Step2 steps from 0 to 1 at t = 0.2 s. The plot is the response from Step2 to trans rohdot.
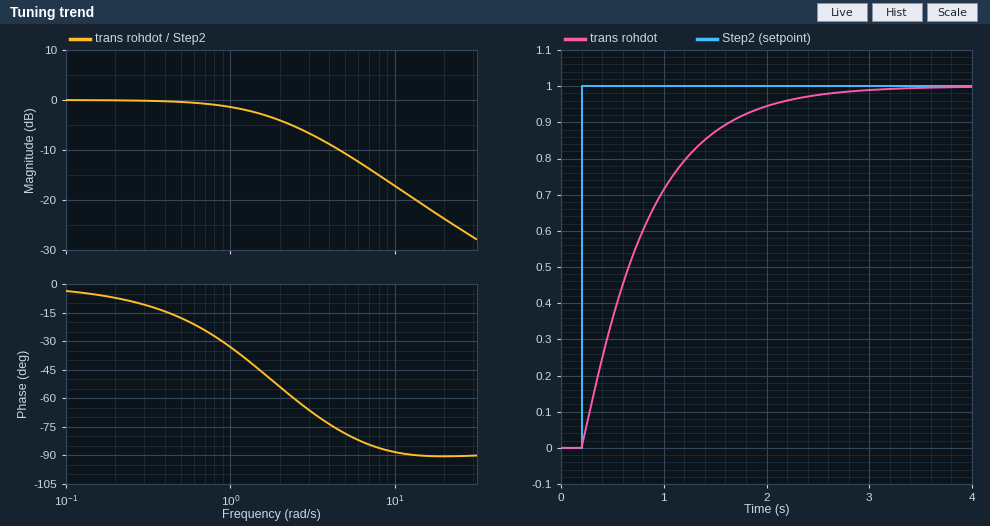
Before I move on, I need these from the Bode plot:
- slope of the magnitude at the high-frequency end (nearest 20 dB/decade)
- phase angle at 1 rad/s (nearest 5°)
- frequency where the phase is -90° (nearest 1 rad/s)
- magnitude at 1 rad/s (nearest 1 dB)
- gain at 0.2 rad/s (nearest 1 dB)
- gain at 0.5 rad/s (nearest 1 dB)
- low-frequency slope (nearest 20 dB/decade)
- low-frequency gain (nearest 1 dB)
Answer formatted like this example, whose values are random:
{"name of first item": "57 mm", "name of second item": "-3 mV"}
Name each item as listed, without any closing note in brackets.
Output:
{"slope of the magnitude at the high-frequency end": "-20 dB/decade", "phase angle at 1 rad/s": "-35°", "frequency where the phase is -90°": "14 rad/s", "magnitude at 1 rad/s": "-1 dB", "gain at 0.2 rad/s": "0 dB", "gain at 0.5 rad/s": "0 dB", "low-frequency slope": "0 dB/decade", "low-frequency gain": "0 dB"}
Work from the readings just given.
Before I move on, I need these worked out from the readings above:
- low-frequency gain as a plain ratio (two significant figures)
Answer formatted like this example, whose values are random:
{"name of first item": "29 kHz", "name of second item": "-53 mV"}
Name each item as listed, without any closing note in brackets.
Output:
{"low-frequency gain as a plain ratio": "1.0"}
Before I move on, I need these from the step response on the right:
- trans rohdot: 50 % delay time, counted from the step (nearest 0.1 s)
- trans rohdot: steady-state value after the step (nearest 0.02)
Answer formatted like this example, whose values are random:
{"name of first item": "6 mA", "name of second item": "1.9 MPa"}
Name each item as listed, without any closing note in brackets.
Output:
{"trans rohdot: 50 % delay time, counted from the step": "0.5 s", "trans rohdot: steady-state value after the step": "1.00"}
